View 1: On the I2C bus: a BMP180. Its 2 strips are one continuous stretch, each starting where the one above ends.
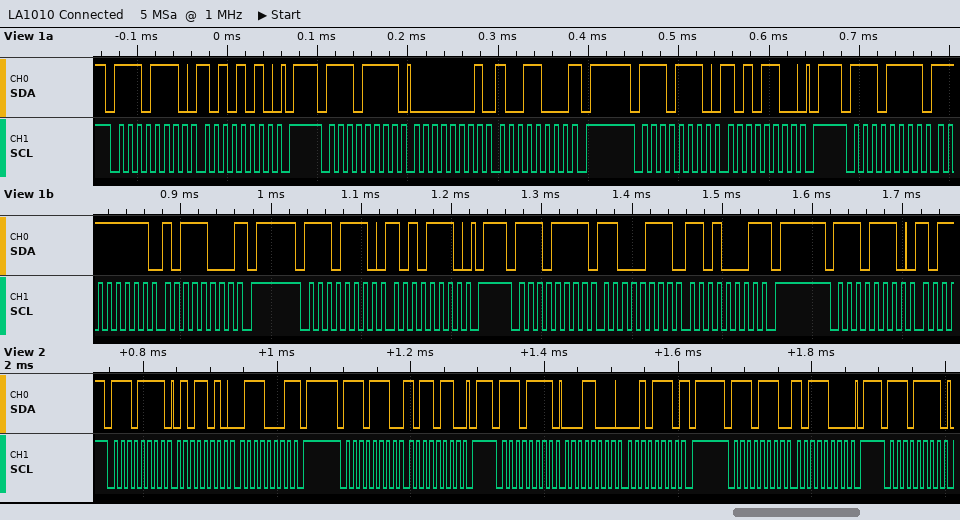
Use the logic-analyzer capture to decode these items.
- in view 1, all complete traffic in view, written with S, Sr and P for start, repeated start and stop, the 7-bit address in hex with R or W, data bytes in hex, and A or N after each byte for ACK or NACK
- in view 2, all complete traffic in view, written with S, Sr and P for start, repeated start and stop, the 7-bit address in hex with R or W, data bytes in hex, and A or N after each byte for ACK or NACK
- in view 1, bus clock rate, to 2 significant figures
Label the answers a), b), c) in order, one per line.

a) S 77W A AA A P S 77R A 01 A 98 N P S 77W A AC A P S 77R A FF A B8 N P S 77W A AE A P S 77R A C7 A D1 N P S 77W A
b) S 77R A 5A A 71 N P S 77W A B6 A P S 77R A 18 A 2E N P S 77W A B8 A P S 77R A
c) 100 kHz
